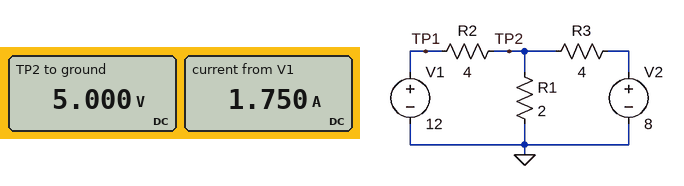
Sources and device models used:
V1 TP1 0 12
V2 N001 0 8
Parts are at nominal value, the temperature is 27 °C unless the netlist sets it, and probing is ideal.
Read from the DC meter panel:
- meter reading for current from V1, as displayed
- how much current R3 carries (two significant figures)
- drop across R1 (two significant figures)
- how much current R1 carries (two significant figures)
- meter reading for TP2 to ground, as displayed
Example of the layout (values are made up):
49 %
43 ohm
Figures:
1.750 A
750 mA
5.0 V
2.5 A
5.000 V
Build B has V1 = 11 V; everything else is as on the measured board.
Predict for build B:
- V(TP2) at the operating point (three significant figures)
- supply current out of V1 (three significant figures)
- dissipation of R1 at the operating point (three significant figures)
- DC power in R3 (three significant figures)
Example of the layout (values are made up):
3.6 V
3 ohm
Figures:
4.75 V
1.56 A
11.3 W
2.64 W
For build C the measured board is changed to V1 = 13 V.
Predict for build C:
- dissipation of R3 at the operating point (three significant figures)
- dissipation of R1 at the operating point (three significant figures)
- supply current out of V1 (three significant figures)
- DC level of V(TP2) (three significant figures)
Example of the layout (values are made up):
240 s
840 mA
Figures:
1.89 W
13.8 W
1.94 A
5.25 V
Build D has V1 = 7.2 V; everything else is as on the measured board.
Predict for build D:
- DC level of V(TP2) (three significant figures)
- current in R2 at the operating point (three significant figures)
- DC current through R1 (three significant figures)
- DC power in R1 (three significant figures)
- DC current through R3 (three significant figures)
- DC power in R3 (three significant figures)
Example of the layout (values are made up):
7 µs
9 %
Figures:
3.80 V
850 mA
1.90 A
7.22 W
1.05 A
4.41 W
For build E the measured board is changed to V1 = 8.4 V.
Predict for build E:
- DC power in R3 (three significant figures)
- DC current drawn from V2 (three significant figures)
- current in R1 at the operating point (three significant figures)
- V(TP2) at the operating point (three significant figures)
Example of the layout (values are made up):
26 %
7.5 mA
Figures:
3.80 W
975 mA
2.05 A
4.10 V
